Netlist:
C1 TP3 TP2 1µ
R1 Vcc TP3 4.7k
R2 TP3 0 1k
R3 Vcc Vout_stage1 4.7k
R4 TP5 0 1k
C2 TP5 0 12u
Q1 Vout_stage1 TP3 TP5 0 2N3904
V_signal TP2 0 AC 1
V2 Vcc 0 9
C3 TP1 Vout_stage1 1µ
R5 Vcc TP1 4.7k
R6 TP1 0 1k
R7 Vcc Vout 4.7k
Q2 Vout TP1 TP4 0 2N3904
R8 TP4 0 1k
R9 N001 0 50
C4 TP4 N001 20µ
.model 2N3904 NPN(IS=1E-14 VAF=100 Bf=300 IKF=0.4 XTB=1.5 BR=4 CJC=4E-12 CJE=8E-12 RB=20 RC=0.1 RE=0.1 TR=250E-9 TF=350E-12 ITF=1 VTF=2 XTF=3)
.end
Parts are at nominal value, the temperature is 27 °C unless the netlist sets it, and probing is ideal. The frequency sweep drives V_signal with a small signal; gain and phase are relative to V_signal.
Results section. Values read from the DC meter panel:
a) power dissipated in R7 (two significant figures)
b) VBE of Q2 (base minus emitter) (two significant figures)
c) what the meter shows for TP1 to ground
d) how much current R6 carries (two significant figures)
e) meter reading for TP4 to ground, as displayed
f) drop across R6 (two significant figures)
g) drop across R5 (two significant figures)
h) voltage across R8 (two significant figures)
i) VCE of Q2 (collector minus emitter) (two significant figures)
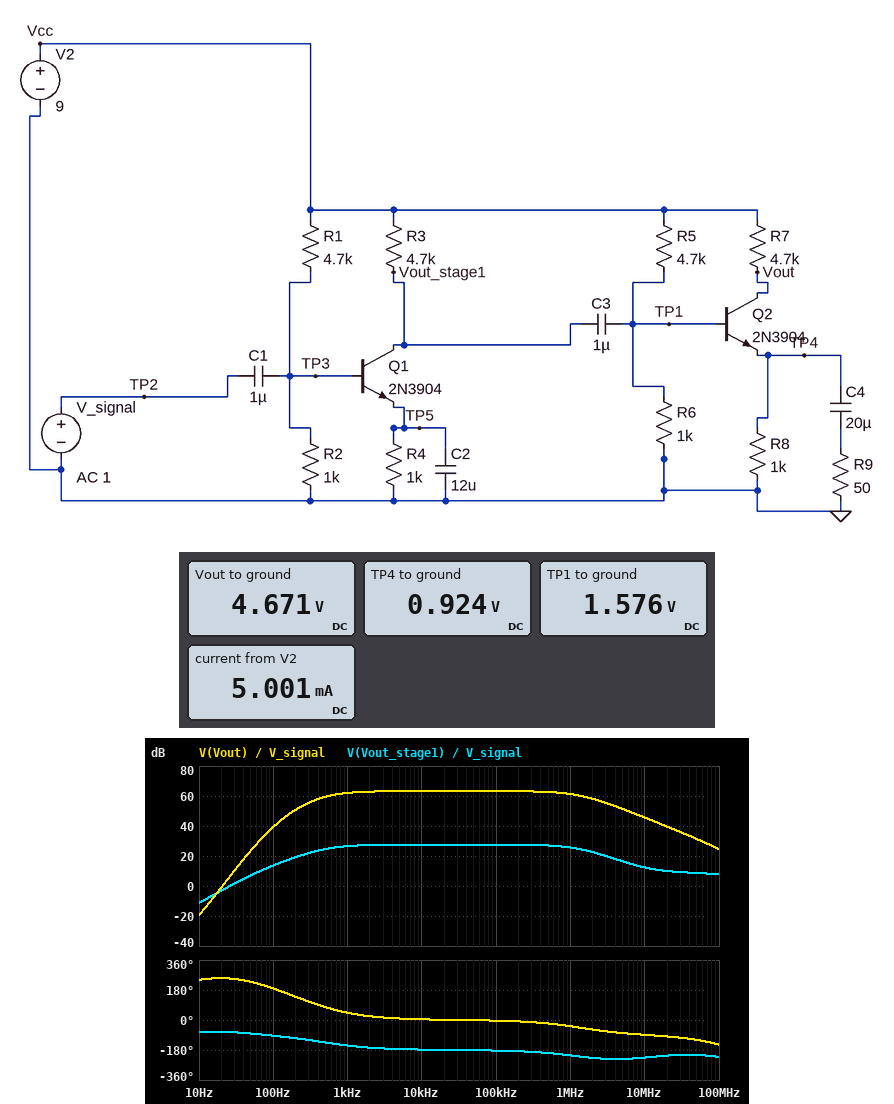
4.0 mW
650 mV
1.576 V
1.6 mA
0.924 V
1.6 V
7.4 V
920 mV
3.7 V
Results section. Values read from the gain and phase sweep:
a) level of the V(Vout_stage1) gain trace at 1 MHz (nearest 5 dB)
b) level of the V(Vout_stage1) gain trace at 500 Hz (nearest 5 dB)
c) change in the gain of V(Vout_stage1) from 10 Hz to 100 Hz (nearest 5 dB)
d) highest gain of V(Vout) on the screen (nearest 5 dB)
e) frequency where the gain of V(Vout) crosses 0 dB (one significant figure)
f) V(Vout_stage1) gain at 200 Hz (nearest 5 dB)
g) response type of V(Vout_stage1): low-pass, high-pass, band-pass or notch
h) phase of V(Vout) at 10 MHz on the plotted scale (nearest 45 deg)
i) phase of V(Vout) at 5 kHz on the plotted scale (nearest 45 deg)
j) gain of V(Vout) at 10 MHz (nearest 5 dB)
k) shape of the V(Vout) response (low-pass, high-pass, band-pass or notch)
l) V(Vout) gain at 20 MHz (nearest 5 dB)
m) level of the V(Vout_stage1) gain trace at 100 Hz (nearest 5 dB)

25 dB
25 dB
25 dB
65 dB
20 Hz
20 dB
band-pass
-90 deg
0 deg
45 dB
band-pass
40 dB
15 dB
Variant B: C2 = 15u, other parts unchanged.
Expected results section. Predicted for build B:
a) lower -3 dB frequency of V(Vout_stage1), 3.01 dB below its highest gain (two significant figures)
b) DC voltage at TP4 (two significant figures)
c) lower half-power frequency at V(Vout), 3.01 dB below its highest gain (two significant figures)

400 Hz
920 mV
500 Hz
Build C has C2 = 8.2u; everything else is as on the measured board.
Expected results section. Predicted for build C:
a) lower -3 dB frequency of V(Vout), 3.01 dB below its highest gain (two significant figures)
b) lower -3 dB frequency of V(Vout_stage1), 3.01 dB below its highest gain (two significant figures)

780 Hz
720 Hz
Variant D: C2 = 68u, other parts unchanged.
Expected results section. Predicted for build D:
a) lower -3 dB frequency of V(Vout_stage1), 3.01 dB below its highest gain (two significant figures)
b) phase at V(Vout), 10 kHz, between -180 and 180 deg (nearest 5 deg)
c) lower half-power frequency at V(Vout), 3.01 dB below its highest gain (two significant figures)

99 Hz
0 deg
280 Hz
